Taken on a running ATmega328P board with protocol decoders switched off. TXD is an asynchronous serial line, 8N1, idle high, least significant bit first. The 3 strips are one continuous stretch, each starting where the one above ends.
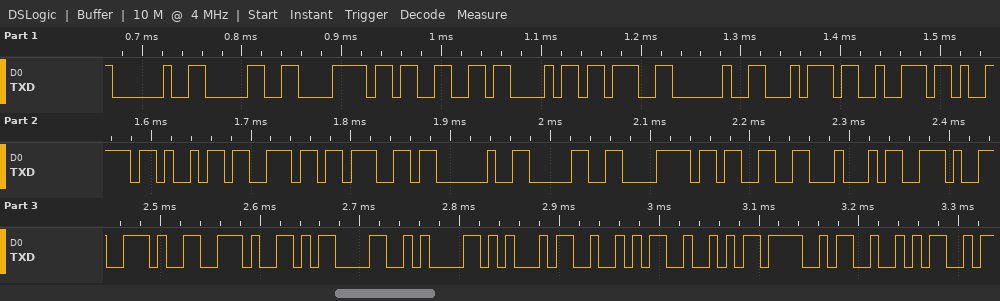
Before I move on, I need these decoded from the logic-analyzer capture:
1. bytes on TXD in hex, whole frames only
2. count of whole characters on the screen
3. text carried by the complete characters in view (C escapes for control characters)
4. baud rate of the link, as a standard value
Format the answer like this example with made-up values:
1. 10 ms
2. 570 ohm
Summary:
1. 20 30 78 33 43 3B 20 74 72 79 69 6E 67 20 30 78 33 44 2E 2E 2E 0D 0A 45 52 52 4F 52
2. 28
3. " 0x3C; trying 0x3D...\r\nERROR"
4. 115200 baud
